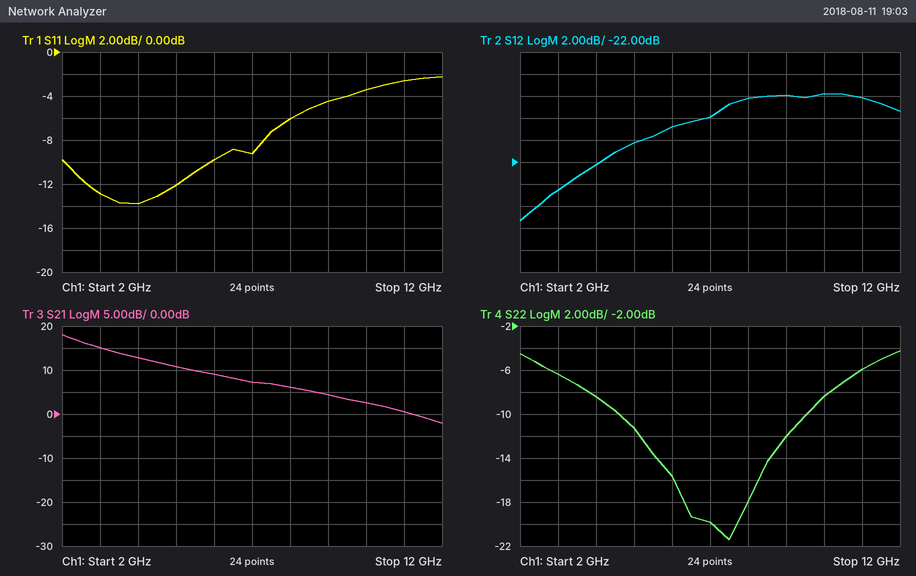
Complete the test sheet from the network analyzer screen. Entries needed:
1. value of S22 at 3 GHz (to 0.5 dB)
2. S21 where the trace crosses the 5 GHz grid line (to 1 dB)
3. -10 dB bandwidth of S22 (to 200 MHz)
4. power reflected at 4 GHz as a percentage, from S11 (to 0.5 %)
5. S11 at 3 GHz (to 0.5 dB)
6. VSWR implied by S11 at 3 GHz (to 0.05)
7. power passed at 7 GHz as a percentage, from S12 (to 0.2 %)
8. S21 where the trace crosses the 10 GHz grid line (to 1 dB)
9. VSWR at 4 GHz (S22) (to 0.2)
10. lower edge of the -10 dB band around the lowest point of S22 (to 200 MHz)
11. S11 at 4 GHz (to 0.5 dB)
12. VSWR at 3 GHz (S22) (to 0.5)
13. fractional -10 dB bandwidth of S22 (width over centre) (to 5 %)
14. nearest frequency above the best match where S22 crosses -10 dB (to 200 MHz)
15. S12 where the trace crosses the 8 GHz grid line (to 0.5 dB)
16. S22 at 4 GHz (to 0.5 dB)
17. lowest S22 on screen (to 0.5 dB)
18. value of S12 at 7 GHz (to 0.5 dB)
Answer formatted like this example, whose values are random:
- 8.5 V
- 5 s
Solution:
- -6.5 dB
- 11 dB
- 5.0 GHz
- 4.0 %
- -13.0 dB
- 1.60
- 1.6 %
- 3 dB
- 2.2
- 4.6 GHz
- -14.0 dB
- 3.0
- 70 %
- 9.6 GHz
- -16.0 dB
- -8.5 dB
- -21.5 dB
- -18.0 dB
